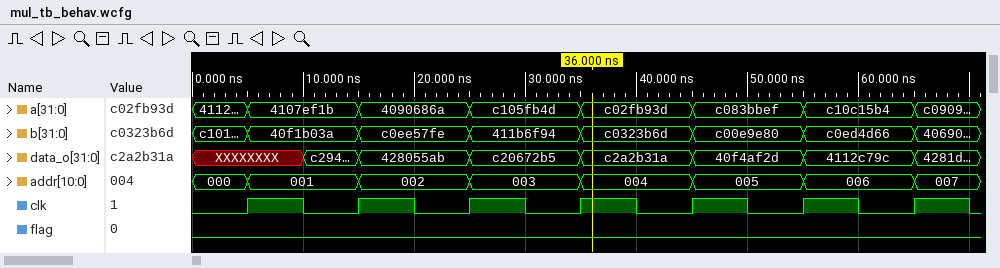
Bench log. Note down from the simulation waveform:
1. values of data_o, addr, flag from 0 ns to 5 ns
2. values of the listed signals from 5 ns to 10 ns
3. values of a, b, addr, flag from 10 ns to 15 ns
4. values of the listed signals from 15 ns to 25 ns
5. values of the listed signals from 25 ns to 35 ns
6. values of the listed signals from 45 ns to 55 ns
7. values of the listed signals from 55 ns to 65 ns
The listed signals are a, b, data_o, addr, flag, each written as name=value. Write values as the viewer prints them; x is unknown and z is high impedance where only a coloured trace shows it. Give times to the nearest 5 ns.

data_o=XXXXXXXX, addr=000, flag=0
a=4107ef1b, b=40f1b03a, data_o=XXXXXXXX, addr=001, flag=0
a=4107ef1b, b=40f1b03a, addr=001, flag=0
a=4090686a, b=c0ee57fe, data_o=428055ab, addr=002, flag=0
a=c105fb4d, b=411b6f94, data_o=c20672b5, addr=003, flag=0
a=c083bbef, b=c00e9e80, data_o=40f4af2d, addr=005, flag=0
a=c10c15b4, b=c0ed4d66, data_o=4112c79c, addr=006, flag=0
